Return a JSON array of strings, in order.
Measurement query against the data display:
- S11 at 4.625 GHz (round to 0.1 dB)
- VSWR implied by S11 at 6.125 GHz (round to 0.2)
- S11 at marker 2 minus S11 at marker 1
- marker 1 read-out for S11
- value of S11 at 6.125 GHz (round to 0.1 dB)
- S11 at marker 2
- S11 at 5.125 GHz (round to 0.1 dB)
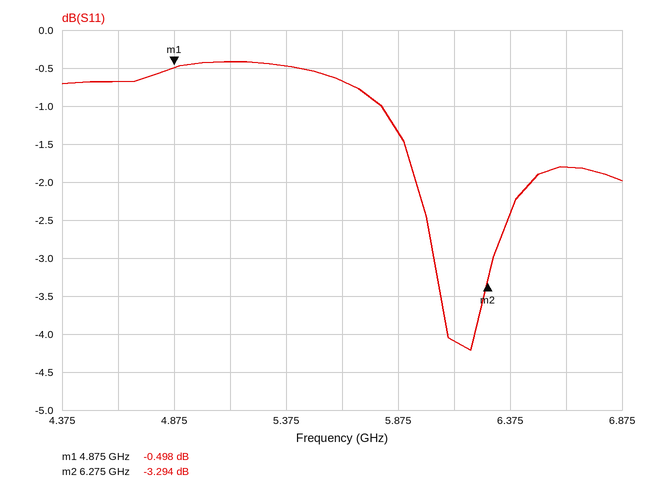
["-0.7 dB", "4.4", "-2.796 dB", "-0.498 dB", "-4.1 dB", "-3.294 dB", "-0.4 dB"]
